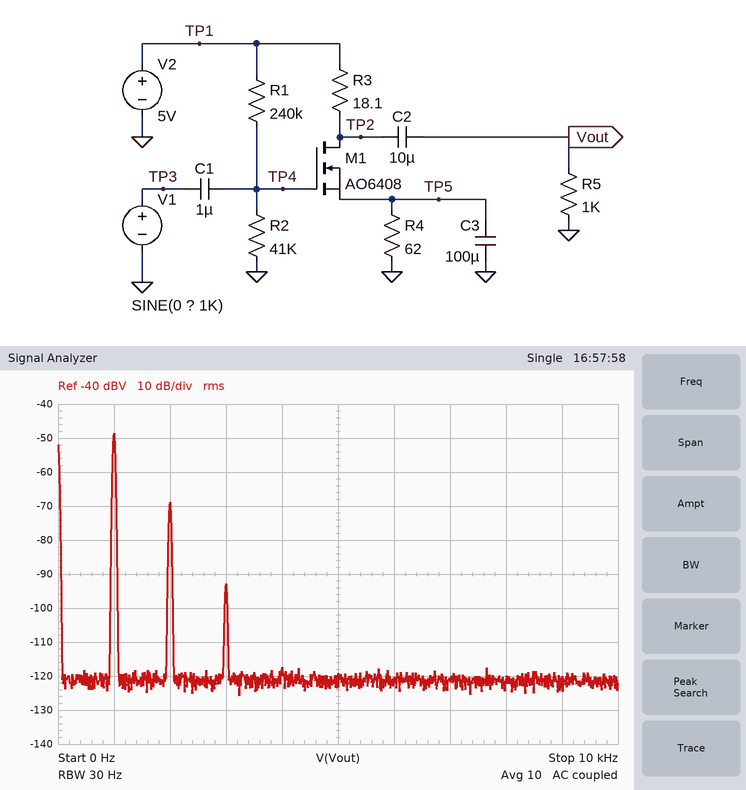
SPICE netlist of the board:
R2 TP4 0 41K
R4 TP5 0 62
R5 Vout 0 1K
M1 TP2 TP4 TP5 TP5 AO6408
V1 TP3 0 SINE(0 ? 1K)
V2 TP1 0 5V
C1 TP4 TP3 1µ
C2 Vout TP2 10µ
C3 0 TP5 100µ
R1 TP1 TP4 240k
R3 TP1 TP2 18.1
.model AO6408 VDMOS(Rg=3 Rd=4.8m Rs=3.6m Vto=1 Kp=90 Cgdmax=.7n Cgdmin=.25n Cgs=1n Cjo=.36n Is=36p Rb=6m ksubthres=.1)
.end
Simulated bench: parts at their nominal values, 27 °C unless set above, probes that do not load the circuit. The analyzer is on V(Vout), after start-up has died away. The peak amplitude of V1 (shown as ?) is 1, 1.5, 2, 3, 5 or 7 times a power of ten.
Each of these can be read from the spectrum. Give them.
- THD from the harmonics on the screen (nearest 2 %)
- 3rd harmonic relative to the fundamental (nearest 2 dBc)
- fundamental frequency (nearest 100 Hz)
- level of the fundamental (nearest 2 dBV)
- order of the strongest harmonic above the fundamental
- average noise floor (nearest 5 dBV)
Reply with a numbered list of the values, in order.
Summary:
1. 10 %
2. -44 dBc
3. 1.0 kHz
4. -48 dBV
5. 2
6. -120 dBV
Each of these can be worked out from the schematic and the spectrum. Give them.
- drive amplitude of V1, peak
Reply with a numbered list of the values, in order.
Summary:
1. 20 mV
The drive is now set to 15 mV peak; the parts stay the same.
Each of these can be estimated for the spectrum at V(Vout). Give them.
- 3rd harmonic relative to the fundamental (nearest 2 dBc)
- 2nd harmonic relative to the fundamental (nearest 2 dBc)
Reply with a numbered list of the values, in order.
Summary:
1. -50 dBc
2. -22 dBc
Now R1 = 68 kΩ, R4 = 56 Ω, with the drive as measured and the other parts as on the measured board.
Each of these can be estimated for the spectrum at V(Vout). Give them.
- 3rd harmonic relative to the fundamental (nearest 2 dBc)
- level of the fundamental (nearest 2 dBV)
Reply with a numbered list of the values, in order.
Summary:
1. -48 dBc
2. -22 dBV
